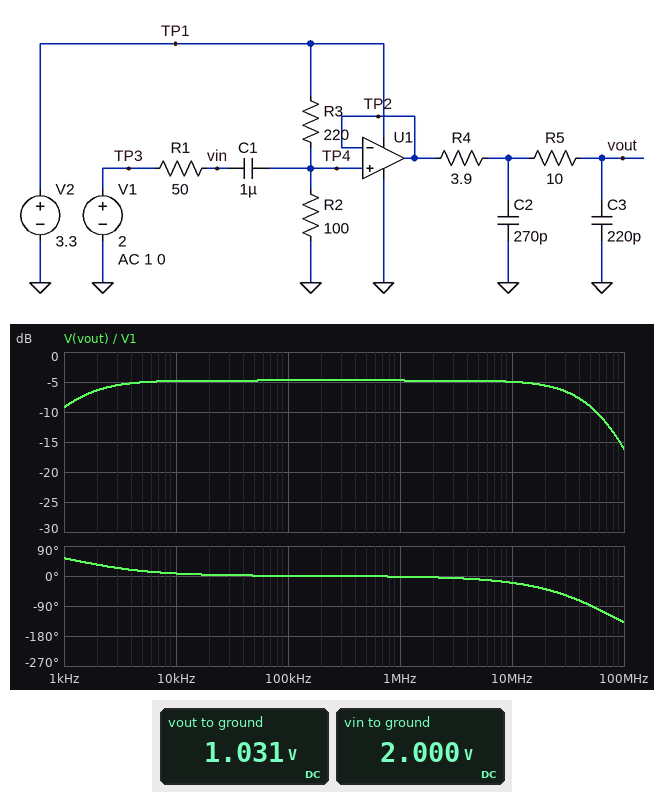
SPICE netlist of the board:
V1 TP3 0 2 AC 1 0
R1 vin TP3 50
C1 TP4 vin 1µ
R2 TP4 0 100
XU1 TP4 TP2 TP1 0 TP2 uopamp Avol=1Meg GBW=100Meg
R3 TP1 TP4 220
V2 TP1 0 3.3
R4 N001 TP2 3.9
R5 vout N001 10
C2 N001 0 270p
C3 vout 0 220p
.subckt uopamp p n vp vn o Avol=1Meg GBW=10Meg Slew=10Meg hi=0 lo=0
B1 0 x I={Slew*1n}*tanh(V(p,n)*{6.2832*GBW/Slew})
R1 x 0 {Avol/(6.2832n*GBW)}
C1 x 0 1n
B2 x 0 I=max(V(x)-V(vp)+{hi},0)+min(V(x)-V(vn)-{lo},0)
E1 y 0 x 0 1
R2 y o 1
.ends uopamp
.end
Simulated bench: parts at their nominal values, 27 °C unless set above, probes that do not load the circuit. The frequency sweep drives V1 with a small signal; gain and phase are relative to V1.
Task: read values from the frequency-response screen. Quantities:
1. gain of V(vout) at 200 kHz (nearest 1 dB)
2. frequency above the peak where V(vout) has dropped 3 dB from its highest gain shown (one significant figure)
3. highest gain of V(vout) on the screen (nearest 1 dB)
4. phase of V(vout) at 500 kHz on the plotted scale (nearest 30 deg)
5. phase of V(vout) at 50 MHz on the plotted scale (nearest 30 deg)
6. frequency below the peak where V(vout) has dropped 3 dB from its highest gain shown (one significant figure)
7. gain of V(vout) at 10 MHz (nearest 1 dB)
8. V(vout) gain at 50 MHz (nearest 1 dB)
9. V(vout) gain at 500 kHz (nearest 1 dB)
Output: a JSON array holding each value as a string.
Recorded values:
["-5 dB", "40 MHz", "-5 dB", "0 deg", "-90 deg", "1 kHz", "-5 dB", "-9 dB", "-5 dB"]
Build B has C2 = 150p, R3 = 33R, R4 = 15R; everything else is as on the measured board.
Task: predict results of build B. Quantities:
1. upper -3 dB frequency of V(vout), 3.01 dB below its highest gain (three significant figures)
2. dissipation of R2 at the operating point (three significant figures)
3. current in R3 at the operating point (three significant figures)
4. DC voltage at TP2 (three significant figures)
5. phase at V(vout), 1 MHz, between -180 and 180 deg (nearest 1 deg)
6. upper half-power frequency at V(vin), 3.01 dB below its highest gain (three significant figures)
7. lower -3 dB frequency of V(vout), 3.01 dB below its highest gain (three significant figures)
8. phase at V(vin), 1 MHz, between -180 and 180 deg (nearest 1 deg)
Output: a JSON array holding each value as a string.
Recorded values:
["21.6 MHz", "61.6 mW", "24.8 mA", "2.48 V", "-3 deg", "2.41 kHz", "2.13 kHz", "0 deg"]
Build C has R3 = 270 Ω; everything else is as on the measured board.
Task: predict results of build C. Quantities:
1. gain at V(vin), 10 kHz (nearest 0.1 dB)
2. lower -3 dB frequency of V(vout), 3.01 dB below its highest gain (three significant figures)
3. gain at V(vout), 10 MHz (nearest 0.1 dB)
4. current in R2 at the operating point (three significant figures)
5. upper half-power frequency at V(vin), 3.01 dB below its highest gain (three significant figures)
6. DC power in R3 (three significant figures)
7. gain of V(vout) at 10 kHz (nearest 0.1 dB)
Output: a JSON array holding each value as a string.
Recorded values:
["-4.4 dB", "1.29 kHz", "-4.8 dB", "8.92 mA", "2.38 kHz", "21.5 mW", "-4.6 dB"]
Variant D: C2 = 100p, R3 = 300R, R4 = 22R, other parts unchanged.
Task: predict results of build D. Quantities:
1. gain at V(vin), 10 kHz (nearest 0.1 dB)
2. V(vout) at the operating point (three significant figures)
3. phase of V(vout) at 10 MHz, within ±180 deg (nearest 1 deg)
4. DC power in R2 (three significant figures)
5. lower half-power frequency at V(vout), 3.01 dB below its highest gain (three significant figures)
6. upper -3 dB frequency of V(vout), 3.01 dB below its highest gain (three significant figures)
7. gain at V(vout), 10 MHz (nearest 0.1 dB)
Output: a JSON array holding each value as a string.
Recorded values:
["-4.3 dB", "825 mV", "-36 deg", "6.81 mW", "1.27 kHz", "17.8 MHz", "-5.6 dB"]
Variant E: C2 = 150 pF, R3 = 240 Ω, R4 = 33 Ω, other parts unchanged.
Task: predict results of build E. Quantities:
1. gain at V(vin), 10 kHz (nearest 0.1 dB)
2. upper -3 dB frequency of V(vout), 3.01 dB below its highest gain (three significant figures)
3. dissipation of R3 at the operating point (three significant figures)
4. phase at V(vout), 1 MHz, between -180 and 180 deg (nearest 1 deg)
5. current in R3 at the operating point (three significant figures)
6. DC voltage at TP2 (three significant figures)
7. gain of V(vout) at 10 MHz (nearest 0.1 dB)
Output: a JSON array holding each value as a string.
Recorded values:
["-4.5 dB", "11.5 MHz", "22.6 mW", "-6 deg", "9.71 mA", "971 mV", "-7.1 dB"]
